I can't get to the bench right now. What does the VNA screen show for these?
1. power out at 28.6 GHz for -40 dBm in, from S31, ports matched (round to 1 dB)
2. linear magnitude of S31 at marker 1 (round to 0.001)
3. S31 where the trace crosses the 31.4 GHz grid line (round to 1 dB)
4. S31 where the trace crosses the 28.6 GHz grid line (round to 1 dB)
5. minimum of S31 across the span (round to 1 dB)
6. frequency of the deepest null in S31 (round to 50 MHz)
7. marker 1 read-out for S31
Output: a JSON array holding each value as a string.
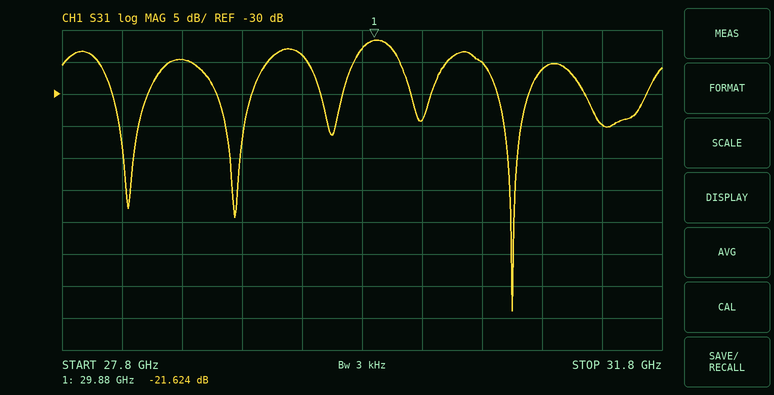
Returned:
["-65 dBm", "0.083", "-35 dB", "-25 dB", "-64 dB", "30.80 GHz", "-21.624 dB"]
